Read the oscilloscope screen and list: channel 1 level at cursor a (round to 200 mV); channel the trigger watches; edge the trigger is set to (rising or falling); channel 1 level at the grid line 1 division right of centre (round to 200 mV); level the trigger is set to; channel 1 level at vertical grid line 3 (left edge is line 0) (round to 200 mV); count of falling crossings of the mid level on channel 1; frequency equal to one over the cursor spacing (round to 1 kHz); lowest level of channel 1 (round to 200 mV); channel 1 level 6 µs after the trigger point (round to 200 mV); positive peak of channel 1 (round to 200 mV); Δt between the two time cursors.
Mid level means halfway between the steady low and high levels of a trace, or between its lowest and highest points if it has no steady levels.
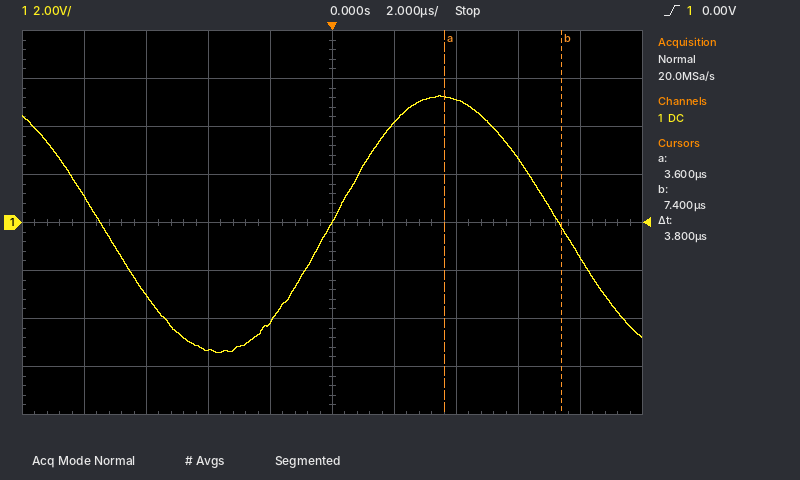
5.2 V
channel 1
rising
4.2 V
0.00 V
-5.4 V
2
263 kHz
-5.4 V
2.6 V
5.2 V
3.8 µs
